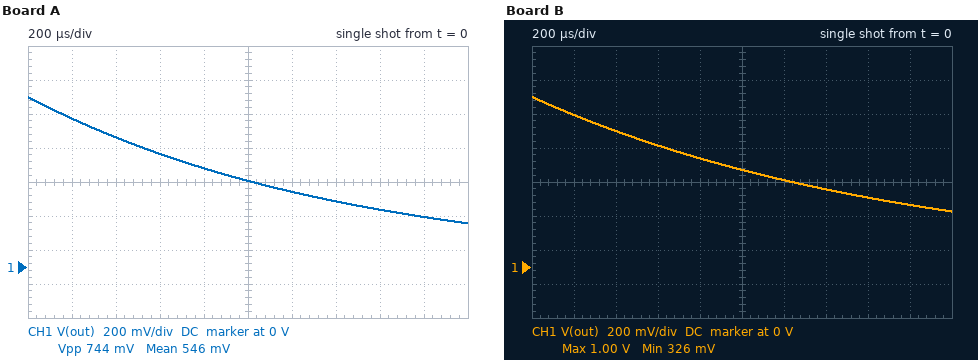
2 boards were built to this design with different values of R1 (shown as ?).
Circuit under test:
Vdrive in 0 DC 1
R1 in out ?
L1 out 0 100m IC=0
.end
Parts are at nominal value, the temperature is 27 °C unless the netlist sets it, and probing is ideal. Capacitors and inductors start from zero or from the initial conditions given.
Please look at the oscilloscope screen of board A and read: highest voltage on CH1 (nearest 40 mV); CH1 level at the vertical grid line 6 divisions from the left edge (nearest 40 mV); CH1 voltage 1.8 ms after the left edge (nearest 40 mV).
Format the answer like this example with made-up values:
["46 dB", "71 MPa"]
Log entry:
["1.00 V", "440 mV", "280 mV"]
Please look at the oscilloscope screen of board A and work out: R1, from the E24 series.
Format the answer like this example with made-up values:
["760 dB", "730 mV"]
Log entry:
["68 Ω"]
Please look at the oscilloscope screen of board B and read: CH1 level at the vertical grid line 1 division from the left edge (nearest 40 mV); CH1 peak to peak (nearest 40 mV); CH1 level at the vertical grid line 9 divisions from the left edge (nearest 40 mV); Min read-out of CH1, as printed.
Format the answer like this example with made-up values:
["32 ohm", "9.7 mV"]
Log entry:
["880 mV", "680 mV", "360 mV", "326 mV"]
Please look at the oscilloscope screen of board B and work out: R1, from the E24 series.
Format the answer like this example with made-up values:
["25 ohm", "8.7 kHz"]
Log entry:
["56 Ω"]
